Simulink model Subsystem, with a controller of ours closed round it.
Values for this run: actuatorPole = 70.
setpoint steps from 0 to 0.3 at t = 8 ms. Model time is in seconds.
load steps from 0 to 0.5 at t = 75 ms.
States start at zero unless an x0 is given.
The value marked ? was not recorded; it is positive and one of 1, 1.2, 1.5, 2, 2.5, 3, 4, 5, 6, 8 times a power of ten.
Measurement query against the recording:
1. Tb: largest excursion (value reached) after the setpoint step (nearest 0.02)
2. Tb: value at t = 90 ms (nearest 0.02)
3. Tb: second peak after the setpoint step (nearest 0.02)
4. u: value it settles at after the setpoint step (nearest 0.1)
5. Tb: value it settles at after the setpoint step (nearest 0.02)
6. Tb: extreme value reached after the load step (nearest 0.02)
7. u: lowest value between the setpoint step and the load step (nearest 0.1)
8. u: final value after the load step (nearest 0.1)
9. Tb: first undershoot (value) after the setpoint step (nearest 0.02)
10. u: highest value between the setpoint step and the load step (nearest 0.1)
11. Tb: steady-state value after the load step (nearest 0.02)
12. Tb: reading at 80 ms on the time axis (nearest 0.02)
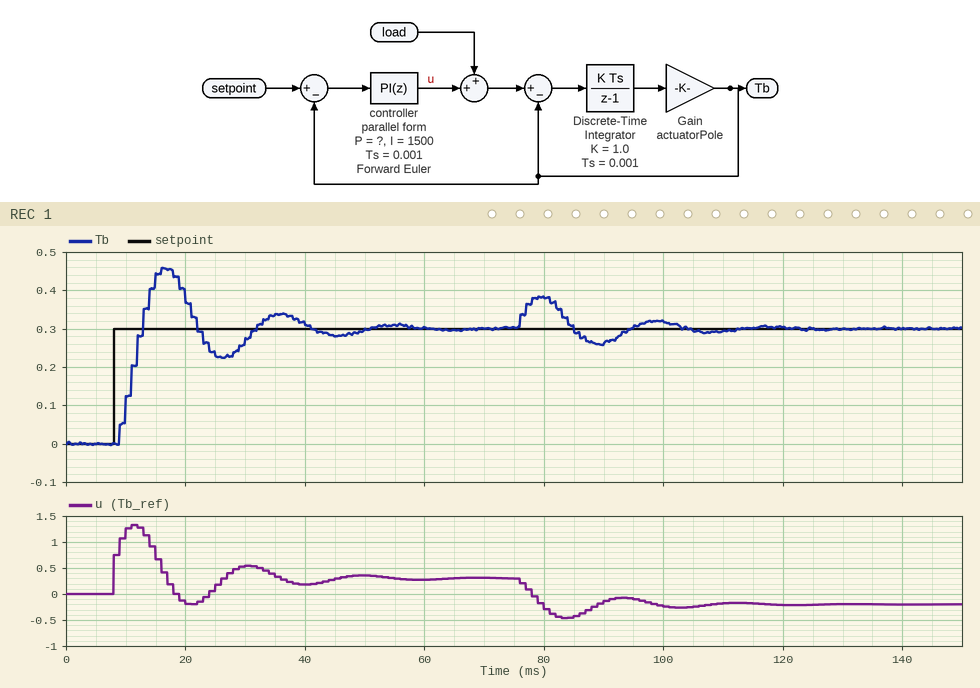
0.46
0.26
0.34
0.3
0.30
0.38
-0.2
-0.2
0.22
1.3
0.30
0.38
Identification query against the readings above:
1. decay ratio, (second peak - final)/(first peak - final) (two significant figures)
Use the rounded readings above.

0.25
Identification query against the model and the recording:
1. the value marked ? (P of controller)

2.5
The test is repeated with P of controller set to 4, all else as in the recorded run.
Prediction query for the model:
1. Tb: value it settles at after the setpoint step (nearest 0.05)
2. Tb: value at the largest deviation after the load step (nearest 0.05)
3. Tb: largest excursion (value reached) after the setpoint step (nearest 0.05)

0.30
0.35
0.40
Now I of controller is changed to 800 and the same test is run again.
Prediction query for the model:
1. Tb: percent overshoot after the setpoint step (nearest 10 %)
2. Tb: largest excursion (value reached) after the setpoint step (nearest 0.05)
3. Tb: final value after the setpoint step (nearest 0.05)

30 %
0.40
0.30
